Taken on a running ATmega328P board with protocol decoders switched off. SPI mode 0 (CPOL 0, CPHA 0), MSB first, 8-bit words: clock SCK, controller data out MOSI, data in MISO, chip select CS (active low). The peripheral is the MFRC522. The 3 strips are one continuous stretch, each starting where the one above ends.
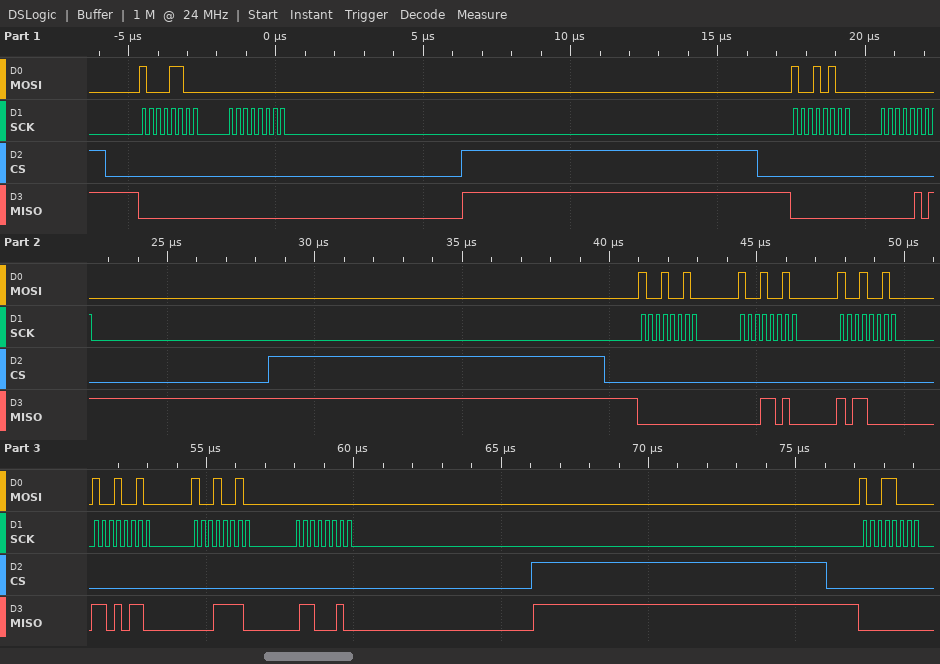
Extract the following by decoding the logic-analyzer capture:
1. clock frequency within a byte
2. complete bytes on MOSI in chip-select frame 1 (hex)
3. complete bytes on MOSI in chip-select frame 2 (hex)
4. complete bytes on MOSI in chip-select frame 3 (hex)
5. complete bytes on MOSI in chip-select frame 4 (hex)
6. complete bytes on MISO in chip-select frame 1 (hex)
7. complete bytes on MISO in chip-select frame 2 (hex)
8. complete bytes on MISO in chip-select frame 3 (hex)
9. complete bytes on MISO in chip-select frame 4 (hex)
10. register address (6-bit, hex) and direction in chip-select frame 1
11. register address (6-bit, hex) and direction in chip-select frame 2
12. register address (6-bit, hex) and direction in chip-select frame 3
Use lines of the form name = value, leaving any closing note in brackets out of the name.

clock frequency within a byte = 4 MHz
complete bytes on MOSI in chip-select frame 1 = 8C 00
complete bytes on MOSI in chip-select frame 2 = 94 00
complete bytes on MOSI in chip-select frame 3 = 92 92 92 92 92 00
complete bytes on MOSI in chip-select frame 4 = 98
complete bytes on MISO in chip-select frame 1 = 00 00
complete bytes on MISO in chip-select frame 2 = 00 05
complete bytes on MISO in chip-select frame 3 = 00 1A B0 D6 1E 62
complete bytes on MISO in chip-select frame 4 = 00
register address (6-bit, hex) and direction in chip-select frame 1 = 0x06 read
register address (6-bit, hex) and direction in chip-select frame 2 = 0x0A read
register address (6-bit, hex) and direction in chip-select frame 3 = 0x09 read
